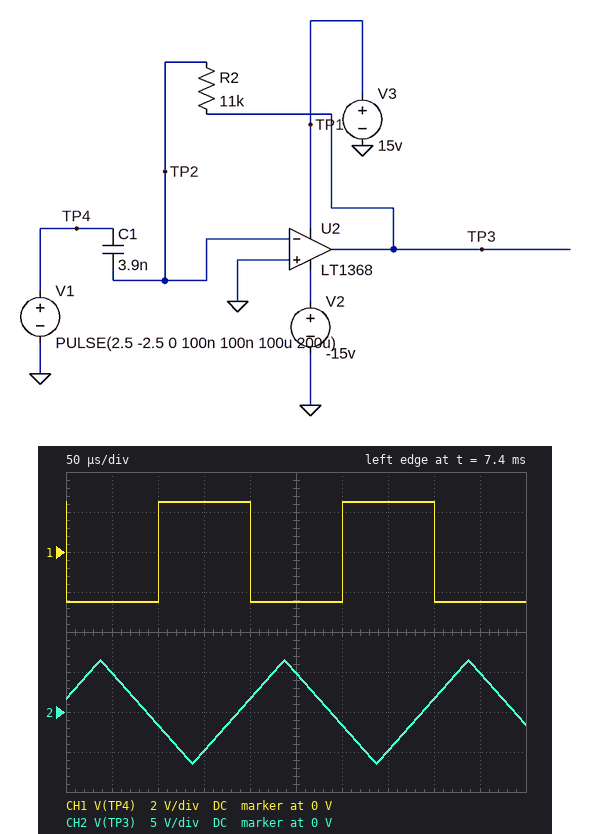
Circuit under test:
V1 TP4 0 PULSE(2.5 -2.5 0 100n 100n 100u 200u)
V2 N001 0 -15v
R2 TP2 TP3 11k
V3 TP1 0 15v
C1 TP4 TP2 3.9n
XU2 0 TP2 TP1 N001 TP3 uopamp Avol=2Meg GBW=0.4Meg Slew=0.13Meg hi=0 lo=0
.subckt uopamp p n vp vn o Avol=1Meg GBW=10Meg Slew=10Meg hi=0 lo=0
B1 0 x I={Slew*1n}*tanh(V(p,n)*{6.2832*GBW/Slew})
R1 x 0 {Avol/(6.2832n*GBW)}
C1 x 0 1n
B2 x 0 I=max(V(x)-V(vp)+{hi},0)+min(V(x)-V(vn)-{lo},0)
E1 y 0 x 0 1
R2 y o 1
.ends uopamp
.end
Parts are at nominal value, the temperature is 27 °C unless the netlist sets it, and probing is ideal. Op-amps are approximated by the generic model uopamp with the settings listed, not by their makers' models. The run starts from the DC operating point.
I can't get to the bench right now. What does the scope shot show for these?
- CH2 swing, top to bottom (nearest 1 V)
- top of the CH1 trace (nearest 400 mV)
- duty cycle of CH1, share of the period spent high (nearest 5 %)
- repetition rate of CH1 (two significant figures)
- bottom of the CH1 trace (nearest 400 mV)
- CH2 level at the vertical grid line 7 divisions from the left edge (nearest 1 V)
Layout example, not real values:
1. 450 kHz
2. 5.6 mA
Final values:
1. 13 V
2. 2.4 V
3. 50 %
4. 5.0 kHz
5. -2.4 V
6. -5 V
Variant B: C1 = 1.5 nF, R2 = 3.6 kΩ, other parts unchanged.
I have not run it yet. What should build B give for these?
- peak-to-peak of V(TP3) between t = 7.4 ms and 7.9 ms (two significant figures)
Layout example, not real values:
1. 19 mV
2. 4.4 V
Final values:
1. 2.6 V
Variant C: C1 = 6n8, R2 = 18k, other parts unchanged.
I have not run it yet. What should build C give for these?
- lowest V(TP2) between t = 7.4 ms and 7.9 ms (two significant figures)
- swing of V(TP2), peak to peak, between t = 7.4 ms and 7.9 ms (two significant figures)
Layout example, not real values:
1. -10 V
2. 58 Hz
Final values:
1. -2.9 V
2. 8.0 V
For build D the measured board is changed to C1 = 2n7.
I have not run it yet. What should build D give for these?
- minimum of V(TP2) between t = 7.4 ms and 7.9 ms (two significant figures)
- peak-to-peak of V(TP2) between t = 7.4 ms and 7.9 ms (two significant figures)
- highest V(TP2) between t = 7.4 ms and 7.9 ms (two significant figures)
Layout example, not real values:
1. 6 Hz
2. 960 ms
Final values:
1. -4.5 V
2. 9.0 V
3. 4.5 V
